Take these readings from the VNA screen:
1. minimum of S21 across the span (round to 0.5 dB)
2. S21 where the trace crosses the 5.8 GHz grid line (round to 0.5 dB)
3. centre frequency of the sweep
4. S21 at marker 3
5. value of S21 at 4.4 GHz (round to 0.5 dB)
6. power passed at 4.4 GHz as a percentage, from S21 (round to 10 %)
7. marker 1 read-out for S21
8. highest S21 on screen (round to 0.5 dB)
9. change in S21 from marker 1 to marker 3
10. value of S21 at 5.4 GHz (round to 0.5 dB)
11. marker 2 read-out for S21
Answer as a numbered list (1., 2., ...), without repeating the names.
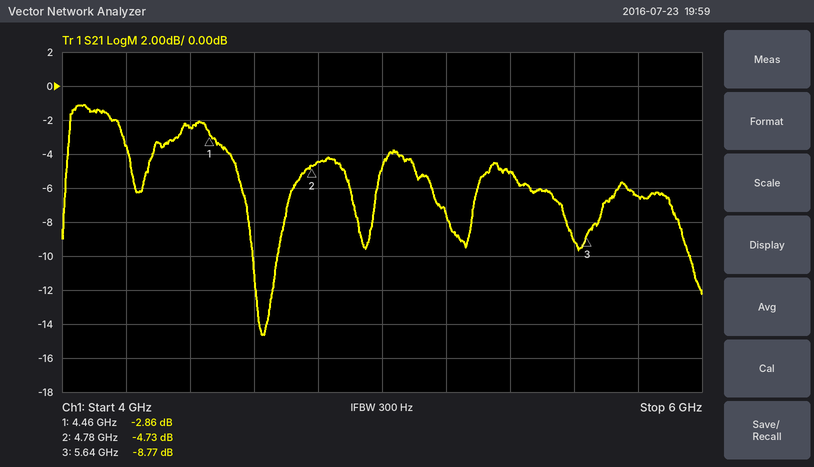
1. -14.5 dB
2. -6.5 dB
3. 5 GHz
4. -8.77 dB
5. -2.5 dB
6. 60 %
7. -2.86 dB
8. -1.0 dB
9. -5.91 dB
10. -5.0 dB
11. -4.73 dB
